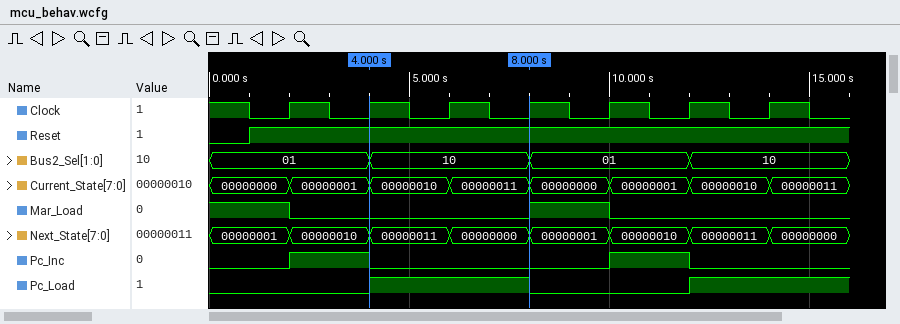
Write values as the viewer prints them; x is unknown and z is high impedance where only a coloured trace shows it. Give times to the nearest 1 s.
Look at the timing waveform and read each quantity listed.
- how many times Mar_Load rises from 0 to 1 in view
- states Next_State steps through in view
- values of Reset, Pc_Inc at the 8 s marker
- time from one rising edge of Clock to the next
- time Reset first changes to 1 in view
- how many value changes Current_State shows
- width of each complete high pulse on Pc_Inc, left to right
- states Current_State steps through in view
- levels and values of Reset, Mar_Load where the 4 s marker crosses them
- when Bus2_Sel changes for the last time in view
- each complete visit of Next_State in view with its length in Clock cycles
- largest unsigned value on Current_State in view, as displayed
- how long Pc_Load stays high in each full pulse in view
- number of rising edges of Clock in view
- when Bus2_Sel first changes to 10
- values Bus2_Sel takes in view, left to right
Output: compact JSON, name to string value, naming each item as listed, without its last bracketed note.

{"how many times Mar_Load rises from 0 to 1 in view": "1", "states Next_State steps through in view": "00000001, 00000010, 00000011, 00000000, 00000001, 00000010, 00000011, 00000000", "values of Reset, Pc_Inc at the 8 s marker": "Reset=1, Pc_Inc=0", "time from one rising edge of Clock to the next": "2 s", "time Reset first changes to 1 in view": "1 s", "how many value changes Current_State shows": "7", "width of each complete high pulse on Pc_Inc, left to right": "2 s, 2 s", "states Current_State steps through in view": "00000000, 00000001, 00000010, 00000011, 00000000, 00000001, 00000010, 00000011", "levels and values of Reset, Mar_Load where the 4 s marker crosses them": "Reset=1, Mar_Load=0", "when Bus2_Sel changes for the last time in view": "12 s", "each complete visit of Next_State in view with its length in Clock cycles": "00000010: 1, 00000011: 1, 00000000: 1, 00000001: 1, 00000010: 1, 00000011: 1", "largest unsigned value on Current_State in view, as displayed": "00000011", "how long Pc_Load stays high in each full pulse in view": "4 s", "number of rising edges of Clock in view": "7", "when Bus2_Sel first changes to 10": "4 s", "values Bus2_Sel takes in view, left to right": "01, 10, 01, 10"}
